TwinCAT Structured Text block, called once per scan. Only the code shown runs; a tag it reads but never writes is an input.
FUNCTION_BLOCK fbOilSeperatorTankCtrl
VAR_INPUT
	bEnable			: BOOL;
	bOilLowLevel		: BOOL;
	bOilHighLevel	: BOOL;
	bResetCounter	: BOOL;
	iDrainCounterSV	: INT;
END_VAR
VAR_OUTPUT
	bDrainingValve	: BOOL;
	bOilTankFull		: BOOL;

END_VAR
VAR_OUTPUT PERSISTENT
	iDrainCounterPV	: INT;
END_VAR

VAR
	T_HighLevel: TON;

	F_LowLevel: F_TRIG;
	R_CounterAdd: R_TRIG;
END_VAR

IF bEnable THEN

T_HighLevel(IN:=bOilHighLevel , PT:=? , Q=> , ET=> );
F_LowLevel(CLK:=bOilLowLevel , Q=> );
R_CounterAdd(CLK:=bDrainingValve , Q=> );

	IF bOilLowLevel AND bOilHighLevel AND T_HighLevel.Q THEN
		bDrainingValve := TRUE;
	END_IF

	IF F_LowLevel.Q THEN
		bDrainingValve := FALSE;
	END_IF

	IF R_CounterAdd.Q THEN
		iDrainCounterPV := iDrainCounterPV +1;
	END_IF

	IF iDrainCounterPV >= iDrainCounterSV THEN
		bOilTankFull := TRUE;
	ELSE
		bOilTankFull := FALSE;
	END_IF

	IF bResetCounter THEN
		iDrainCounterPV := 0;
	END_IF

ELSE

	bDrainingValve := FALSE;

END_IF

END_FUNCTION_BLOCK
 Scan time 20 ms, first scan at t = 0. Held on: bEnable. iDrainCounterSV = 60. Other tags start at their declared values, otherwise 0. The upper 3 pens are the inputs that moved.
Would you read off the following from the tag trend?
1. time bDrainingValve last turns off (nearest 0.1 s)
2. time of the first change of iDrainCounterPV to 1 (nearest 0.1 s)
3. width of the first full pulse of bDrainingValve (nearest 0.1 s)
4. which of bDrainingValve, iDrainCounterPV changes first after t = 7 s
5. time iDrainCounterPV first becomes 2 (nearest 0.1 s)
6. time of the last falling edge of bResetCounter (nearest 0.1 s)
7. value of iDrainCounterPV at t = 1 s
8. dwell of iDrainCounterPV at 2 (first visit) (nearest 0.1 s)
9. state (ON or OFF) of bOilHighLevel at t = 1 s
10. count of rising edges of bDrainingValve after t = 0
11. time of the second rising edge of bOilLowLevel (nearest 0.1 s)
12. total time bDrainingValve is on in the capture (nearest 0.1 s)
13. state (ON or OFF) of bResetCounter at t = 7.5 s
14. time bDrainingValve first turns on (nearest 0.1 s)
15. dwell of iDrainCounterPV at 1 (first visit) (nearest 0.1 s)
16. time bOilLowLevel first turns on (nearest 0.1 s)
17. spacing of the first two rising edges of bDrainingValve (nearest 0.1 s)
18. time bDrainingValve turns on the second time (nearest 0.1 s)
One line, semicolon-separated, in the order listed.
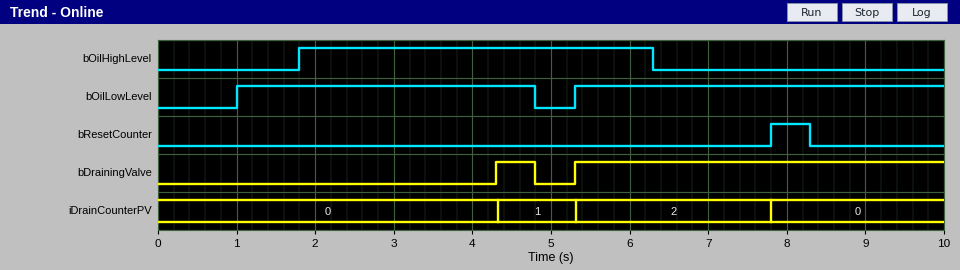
4.8 s; 4.3 s; 0.5 s; iDrainCounterPV; 5.3 s; 8.3 s; 0; 2.5 s; OFF; 2; 5.3 s; 5.2 s; OFF; 4.3 s; 1.0 s; 1.0 s; 1.0 s; 5.3 s
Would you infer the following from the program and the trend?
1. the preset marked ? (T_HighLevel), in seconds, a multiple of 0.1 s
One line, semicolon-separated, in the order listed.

2.5 s
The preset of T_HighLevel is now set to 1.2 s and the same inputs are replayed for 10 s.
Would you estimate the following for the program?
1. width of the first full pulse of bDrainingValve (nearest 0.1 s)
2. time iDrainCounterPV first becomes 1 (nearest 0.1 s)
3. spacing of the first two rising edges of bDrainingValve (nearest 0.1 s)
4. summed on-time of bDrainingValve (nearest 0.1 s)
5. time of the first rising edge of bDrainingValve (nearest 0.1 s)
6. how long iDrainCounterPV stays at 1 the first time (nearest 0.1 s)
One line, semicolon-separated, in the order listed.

1.8 s; 3.0 s; 2.3 s; 6.5 s; 3.0 s; 2.3 s
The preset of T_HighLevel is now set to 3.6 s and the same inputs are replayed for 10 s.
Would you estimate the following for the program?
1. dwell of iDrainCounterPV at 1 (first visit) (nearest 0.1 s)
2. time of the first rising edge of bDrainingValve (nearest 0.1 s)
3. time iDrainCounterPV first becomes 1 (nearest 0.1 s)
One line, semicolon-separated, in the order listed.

2.4 s; 5.4 s; 5.4 s
